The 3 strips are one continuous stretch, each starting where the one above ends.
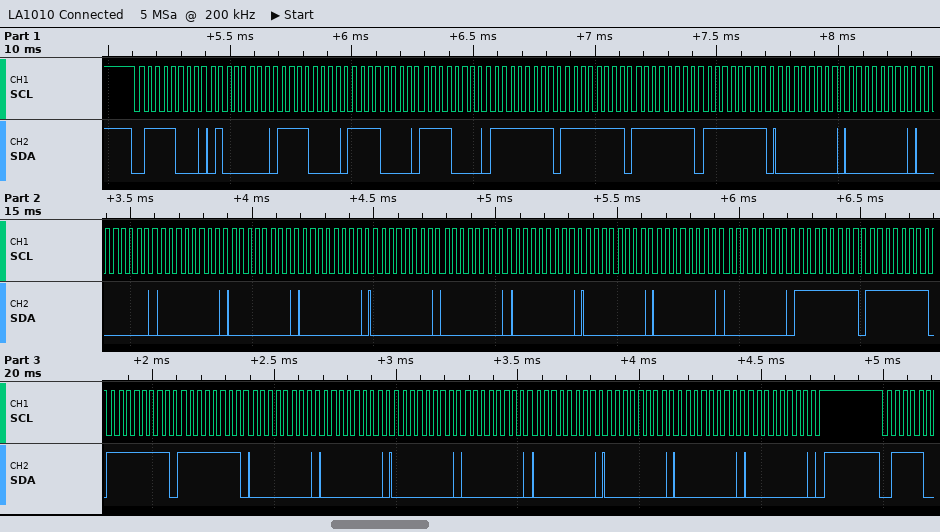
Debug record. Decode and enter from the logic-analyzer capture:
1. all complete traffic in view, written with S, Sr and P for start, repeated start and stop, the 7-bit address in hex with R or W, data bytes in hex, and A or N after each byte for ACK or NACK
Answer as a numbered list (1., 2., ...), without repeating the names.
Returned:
1. S 3CW A 40 A F0 A F0 A F0 A FF A FF A FF A FF A 00 A 00 A 00 A 00 A 00 A 00 A 00 A 00 A 00 A 00 A 00 A 00 A FF A FF A FF A FF A 00 A 00 A 00 A 00 A 00 A 00 A 00 A 00 A P
